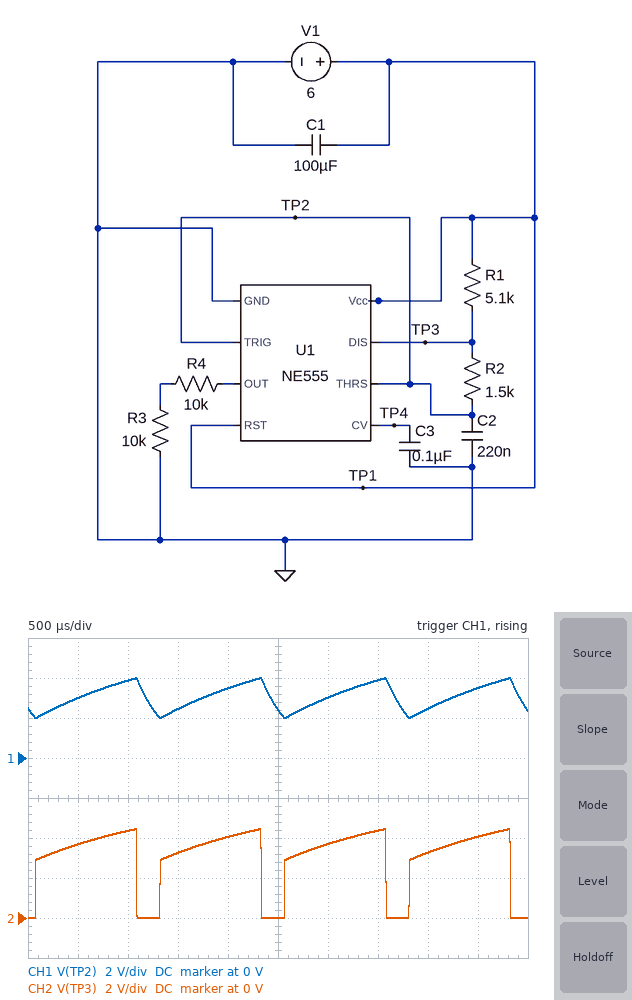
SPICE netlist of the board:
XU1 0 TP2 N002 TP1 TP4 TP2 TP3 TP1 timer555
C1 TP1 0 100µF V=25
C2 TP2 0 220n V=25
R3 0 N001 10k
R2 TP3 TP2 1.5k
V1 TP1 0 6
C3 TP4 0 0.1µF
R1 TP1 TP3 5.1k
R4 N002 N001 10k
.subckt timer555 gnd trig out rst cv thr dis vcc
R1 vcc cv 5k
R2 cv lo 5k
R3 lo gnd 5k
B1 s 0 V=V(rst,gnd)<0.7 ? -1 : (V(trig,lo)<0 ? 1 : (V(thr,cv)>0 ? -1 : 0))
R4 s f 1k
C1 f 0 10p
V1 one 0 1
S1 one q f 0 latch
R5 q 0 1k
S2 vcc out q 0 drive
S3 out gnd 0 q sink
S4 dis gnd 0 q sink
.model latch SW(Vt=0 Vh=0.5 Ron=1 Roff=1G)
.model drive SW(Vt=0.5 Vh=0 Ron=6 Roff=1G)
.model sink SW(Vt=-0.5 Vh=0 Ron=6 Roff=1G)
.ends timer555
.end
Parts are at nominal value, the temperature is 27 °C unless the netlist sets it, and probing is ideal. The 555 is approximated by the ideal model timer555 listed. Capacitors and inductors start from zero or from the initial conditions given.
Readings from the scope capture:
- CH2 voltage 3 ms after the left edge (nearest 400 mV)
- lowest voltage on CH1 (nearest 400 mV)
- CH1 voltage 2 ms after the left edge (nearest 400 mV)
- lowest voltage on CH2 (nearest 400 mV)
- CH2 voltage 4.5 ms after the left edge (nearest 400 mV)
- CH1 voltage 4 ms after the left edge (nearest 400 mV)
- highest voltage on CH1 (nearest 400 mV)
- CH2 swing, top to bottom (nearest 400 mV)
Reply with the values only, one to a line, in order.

3.6 V
2.0 V
3.6 V
0 V
4.0 V
2.4 V
4.0 V
4.4 V
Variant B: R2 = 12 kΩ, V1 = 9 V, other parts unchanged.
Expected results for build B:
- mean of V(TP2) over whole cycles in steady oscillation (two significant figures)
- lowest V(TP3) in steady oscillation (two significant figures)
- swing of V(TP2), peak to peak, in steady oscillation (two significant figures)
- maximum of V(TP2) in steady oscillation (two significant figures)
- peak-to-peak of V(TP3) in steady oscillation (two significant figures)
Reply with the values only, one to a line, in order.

4.5 V
12 mV
3.0 V
6.0 V
8.1 V
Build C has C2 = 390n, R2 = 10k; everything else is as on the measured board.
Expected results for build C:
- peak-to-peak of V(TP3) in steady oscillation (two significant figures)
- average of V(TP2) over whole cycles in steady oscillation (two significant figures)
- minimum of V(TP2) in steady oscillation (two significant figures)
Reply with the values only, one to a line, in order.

5.3 V
3.0 V
2.0 V
